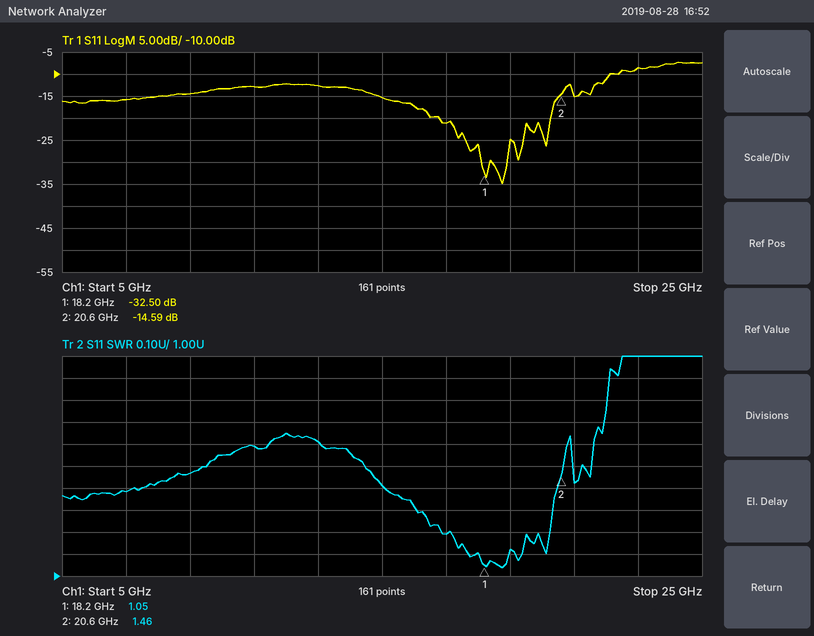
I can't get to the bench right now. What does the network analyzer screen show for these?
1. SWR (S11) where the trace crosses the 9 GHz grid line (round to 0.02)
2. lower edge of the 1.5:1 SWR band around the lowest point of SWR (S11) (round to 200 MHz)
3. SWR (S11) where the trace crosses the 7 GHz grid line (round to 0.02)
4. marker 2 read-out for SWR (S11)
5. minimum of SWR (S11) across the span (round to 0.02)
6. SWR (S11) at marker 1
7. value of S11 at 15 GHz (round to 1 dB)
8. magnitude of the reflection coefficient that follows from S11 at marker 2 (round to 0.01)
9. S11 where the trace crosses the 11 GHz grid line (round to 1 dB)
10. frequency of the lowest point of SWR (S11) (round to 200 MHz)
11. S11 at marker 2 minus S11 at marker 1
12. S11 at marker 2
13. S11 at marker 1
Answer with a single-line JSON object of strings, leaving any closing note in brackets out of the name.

{"SWR (S11) where the trace crosses the 9 GHz grid line": "1.46", "lower edge of the 1.5:1 SWR band around the lowest point of SWR (S11)": "14.4 GHz", "SWR (S11) where the trace crosses the 7 GHz grid line": "1.38", "marker 2 read-out for SWR": "1.46", "minimum of SWR (S11) across the span": "1.04", "SWR (S11) at marker 1": "1.05", "value of S11 at 15 GHz": "-15 dB", "magnitude of the reflection coefficient that follows from S11 at marker 2": "0.19", "S11 where the trace crosses the 11 GHz grid line": "-13 dB", "frequency of the lowest point of SWR (S11)": "18.8 GHz", "S11 at marker 2 minus S11 at marker 1": "17.91 dB", "S11 at marker 2": "-14.59 dB", "S11 at marker 1": "-32.50 dB"}
